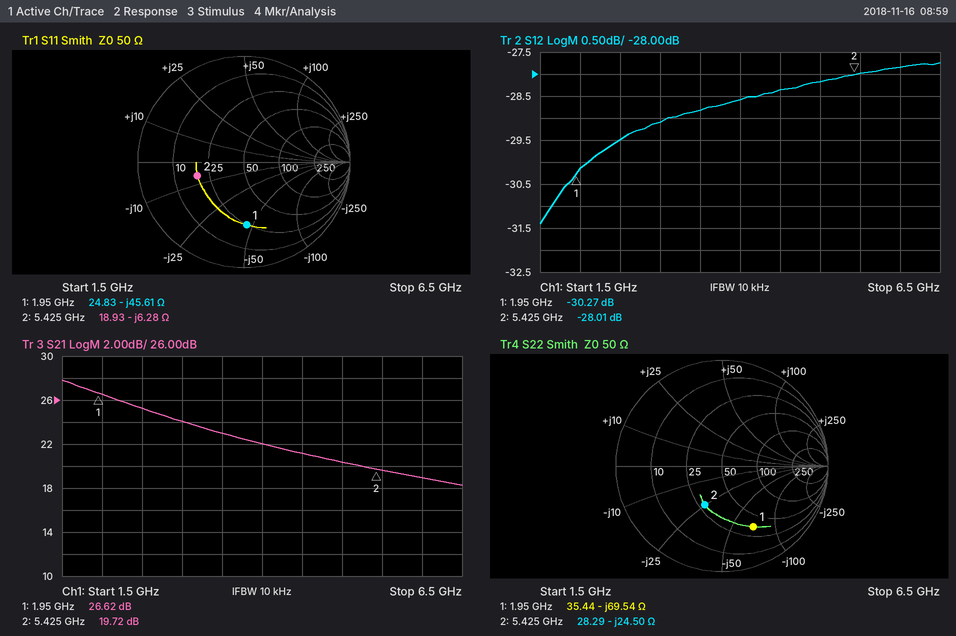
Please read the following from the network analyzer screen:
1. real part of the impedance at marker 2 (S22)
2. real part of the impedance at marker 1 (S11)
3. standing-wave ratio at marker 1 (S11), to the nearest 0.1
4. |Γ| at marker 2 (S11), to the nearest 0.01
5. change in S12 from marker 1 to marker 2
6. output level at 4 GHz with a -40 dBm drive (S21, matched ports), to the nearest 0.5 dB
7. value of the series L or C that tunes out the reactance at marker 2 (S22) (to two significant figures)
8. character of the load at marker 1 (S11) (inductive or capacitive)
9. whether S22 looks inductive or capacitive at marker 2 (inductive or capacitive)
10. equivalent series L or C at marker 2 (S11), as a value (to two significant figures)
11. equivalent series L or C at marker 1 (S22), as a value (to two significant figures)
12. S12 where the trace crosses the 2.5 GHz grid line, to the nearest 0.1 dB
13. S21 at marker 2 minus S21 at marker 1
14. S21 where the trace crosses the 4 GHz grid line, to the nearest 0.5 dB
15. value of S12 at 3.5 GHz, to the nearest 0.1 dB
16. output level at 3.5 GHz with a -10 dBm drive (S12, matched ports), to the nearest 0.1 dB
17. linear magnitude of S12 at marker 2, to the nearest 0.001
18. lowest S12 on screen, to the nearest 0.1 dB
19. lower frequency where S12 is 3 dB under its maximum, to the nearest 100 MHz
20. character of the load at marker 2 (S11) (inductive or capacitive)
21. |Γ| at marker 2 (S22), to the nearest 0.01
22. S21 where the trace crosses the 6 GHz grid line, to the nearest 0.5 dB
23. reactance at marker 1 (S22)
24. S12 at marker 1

28.29 Ω
24.83 Ω
3.9
0.46
2.26 dB
-18.0 dBm
720 pH
capacitive
capacitive
4.7 pF
1.2 pF
-29.5 dB
-6.90 dB
22.0 dB
-28.8 dB
-38.8 dBm
0.040
-31.4 dB
1.7 GHz
capacitive
0.40
19.0 dB
-69.54 Ω
-30.27 dB
